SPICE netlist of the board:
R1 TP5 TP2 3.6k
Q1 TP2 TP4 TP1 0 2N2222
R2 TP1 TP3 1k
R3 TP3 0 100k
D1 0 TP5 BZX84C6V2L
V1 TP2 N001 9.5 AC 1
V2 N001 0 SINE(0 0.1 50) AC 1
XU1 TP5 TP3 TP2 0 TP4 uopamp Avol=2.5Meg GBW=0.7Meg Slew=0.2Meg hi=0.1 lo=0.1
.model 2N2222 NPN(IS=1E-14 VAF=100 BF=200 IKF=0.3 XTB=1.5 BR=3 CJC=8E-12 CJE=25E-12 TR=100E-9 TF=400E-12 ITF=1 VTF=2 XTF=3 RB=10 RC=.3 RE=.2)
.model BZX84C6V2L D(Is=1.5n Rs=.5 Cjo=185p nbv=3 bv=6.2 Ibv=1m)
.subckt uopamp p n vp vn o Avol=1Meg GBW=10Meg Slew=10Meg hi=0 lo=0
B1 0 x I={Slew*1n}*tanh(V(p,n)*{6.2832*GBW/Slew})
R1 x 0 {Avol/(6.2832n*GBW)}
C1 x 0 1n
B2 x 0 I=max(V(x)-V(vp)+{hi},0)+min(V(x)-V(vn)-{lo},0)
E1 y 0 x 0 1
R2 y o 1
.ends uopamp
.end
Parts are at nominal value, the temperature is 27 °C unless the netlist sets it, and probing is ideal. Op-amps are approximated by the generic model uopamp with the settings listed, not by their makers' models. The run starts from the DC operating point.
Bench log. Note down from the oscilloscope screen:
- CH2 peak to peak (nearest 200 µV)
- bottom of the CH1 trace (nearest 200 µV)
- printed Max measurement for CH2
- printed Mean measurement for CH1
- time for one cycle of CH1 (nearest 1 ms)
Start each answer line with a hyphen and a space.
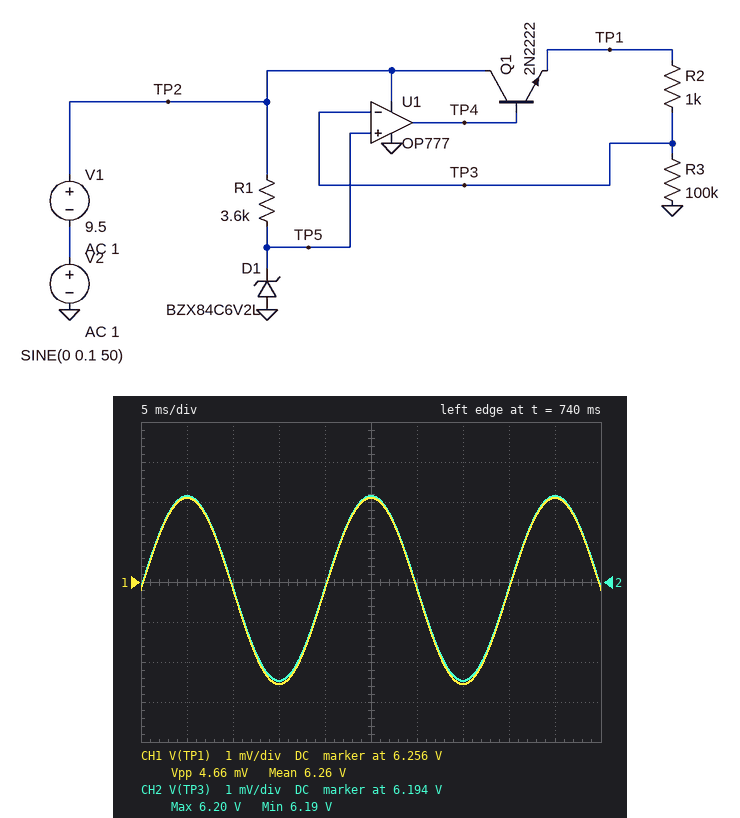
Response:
- 4.6 mV
- 6.2534 V
- 6.20 V
- 6.26 V
- 20 ms
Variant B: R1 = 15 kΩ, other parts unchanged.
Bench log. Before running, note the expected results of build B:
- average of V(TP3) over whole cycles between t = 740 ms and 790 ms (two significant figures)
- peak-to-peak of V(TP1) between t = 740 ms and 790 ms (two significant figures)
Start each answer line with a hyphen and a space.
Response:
- 6.1 V
- 4.5 mV
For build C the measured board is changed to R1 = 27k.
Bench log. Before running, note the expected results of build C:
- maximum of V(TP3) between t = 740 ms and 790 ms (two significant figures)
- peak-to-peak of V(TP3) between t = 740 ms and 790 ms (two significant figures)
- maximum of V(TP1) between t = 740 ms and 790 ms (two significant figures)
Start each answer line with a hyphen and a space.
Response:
- 6.0 V
- 4.4 mV
- 6.1 V
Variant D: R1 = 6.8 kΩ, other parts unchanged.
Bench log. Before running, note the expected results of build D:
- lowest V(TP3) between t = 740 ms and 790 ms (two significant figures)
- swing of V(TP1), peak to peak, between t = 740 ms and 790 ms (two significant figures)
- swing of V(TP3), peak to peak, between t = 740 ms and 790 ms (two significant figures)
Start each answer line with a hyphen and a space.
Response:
- 6.1 V
- 4.6 mV
- 4.5 mV
